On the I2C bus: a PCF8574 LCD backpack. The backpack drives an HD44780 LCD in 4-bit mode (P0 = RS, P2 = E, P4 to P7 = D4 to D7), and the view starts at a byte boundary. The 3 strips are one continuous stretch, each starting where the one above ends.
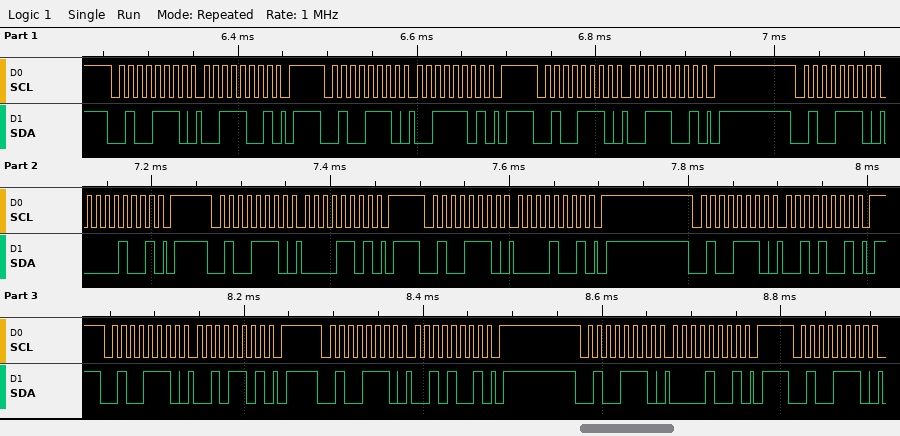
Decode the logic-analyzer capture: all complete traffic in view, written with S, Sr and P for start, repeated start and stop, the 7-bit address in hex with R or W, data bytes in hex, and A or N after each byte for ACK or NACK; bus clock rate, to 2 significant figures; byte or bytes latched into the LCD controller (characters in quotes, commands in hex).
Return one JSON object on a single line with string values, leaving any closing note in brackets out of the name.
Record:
{"all complete traffic in view, written with S, Sr and P for start, repeated start and stop, the 7-bit address in hex with R or W, data bytes in hex, and A or N after each byte for ACK or NACK": "S 27W A 39 A P S 27W A 3D A P S 27W A 39 A P S 27W A 09 A P S 27W A 0D A P S 27W A 09 A P S 27W A 29 A P S 27W A 2D A P S 27W A 29 A P S 27W A 09 A P S 27W A", "bus clock rate, to 2 significant figures": "100 kHz", "byte or bytes latched into the LCD controller": "'0'"}
